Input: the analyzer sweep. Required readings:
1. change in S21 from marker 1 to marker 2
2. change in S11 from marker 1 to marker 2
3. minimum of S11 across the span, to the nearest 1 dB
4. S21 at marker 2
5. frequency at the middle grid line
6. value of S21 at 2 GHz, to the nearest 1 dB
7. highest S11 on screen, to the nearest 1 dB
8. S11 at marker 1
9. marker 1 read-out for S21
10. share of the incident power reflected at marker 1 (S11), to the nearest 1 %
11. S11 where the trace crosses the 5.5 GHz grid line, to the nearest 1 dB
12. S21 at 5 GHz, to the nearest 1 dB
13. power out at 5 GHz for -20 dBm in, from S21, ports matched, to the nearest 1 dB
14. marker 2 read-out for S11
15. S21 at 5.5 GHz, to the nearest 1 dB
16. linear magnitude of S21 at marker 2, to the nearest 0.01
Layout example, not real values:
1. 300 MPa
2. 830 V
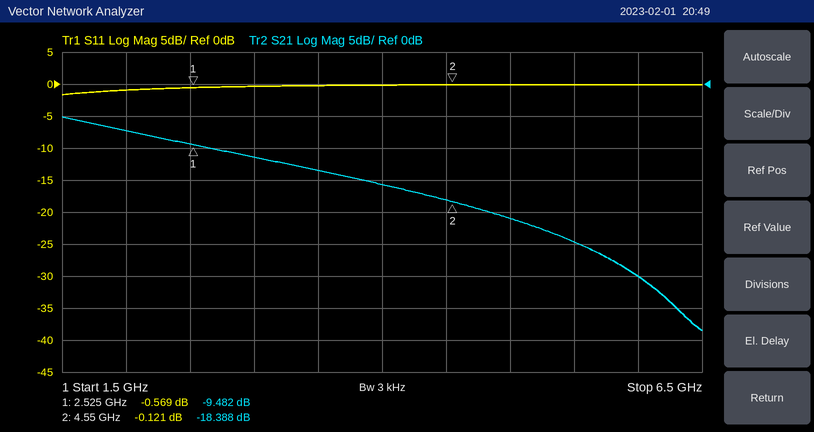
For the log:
1. -8.906 dB
2. 0.448 dB
3. -2 dB
4. -18.388 dB
5. 4 GHz
6. -7 dB
7. 0 dB
8. -0.569 dB
9. -9.482 dB
10. 88 %
11. 0 dB
12. -21 dB
13. -41 dBm
14. -0.121 dB
15. -25 dB
16. 0.12
